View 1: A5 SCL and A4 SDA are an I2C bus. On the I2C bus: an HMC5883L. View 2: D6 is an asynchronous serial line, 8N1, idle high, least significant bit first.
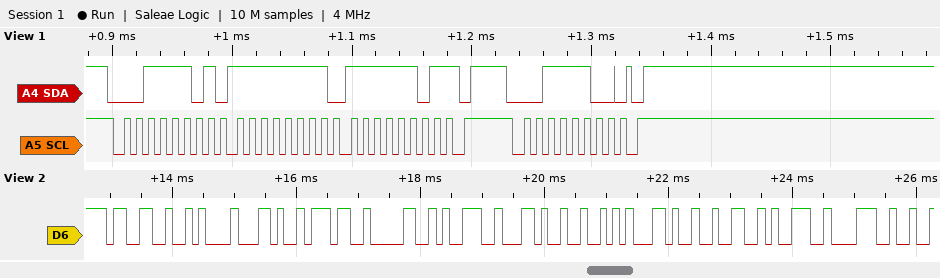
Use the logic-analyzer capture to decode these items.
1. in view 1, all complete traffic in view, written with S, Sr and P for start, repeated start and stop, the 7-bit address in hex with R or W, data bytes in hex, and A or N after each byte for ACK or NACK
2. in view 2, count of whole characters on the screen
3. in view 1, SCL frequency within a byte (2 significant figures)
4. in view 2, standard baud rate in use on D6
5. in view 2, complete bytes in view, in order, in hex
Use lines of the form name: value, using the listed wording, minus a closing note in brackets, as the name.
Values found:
in view 1, all complete traffic in view, written with S, Sr and P for start, repeated start and stop, the 7-bit address in hex with R or W, data bytes in hex, and A or N after each byte for ACK or NACK: S 1ER A FF A FD N P S 1EW A P
in view 2, count of whole characters on the screen: 12
in view 1, SCL frequency within a byte: 100 kHz
in view 2, standard baud rate in use on D6: 9600 baud
in view 2, complete bytes in view, in order, in hex: 33 0A 2C 37 30 39 2C 52 2C 32 39 38
